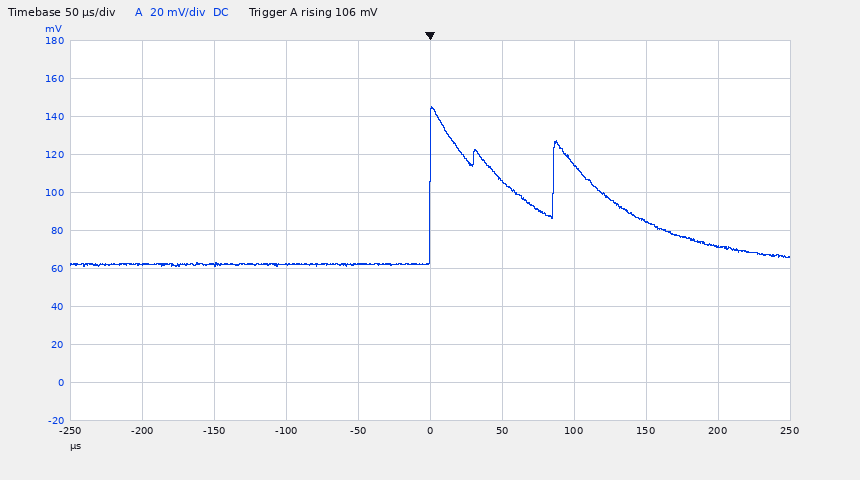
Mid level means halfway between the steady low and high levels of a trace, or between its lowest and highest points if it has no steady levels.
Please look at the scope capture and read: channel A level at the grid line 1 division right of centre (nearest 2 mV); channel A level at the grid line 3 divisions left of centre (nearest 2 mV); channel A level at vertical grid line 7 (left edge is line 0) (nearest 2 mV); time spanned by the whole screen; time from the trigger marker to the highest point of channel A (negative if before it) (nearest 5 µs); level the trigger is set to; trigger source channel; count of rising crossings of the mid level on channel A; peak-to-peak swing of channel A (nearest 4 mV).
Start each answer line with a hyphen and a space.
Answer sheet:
- 106 mV
- 62 mV
- 114 mV
- 500 µs
- 0 µs
- 106 mV
- channel A
- 2
- 84 mV
